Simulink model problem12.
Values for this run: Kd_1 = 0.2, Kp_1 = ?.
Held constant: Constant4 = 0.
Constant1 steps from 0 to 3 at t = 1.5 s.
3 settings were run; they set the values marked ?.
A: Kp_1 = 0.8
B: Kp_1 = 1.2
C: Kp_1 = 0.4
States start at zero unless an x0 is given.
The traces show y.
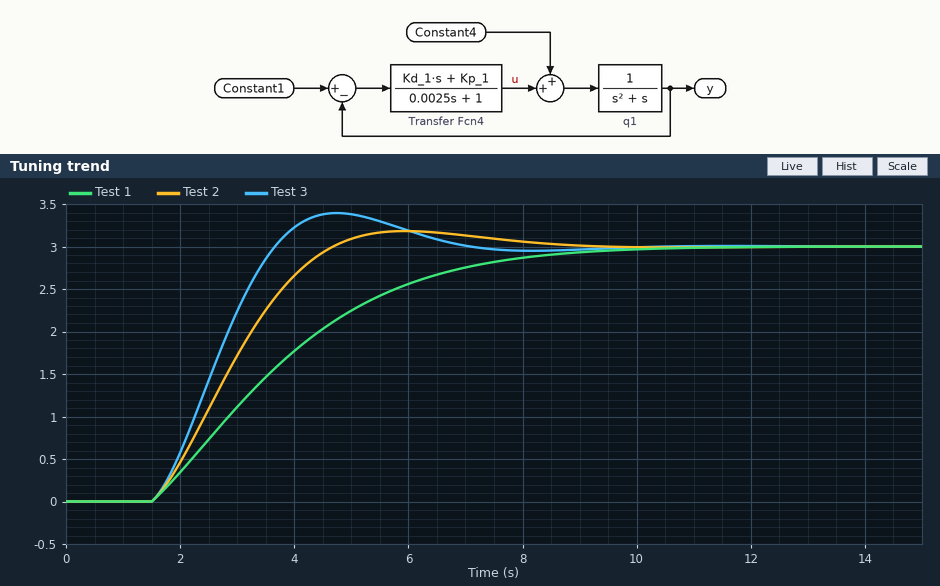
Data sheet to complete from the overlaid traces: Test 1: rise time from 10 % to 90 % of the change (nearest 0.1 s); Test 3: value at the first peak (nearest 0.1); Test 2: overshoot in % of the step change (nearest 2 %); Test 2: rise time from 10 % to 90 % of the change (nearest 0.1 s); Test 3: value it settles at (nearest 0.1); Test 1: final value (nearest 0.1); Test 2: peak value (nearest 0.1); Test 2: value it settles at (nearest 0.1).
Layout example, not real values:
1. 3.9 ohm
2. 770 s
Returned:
1. 4.7 s
2. 3.4
3. 6 %
4. 2.2 s
5. 3.0
6. 3.0
7. 3.2
8. 3.0
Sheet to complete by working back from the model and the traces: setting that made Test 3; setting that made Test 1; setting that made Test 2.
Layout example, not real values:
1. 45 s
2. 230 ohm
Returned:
1. B
2. C
3. A
